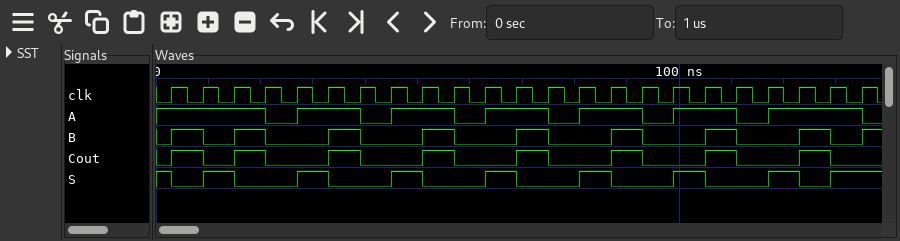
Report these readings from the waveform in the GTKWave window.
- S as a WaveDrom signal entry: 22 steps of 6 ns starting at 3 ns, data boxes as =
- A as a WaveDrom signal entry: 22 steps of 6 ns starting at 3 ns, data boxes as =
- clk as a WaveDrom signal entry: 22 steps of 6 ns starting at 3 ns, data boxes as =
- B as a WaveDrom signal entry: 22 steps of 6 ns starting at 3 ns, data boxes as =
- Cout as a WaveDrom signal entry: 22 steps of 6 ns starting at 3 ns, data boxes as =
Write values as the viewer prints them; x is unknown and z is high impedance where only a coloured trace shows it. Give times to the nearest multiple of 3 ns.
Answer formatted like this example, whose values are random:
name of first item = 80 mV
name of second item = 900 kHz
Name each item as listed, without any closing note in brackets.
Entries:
S as a WaveDrom signal entry: 22 steps of 6 ns starting at 3 ns, data boxes as = = {name: 'S', wave: '010.10.10.10.10.10.101'}
A as a WaveDrom signal entry: 22 steps of 6 ns starting at 3 ns, data boxes as = = {name: 'A', wave: '1..01.01.01.01.01.01..'}
clk as a WaveDrom signal entry: 22 steps of 6 ns starting at 3 ns, data boxes as = = {name: 'clk', wave: 'p.....................'}
B as a WaveDrom signal entry: 22 steps of 6 ns starting at 3 ns, data boxes as = = {name: 'B', wave: '1010.10.10.10.10.10.10'}
Cout as a WaveDrom signal entry: 22 steps of 6 ns starting at 3 ns, data boxes as = = {name: 'Cout', wave: '1010.10.10.10.10.10.10'}
